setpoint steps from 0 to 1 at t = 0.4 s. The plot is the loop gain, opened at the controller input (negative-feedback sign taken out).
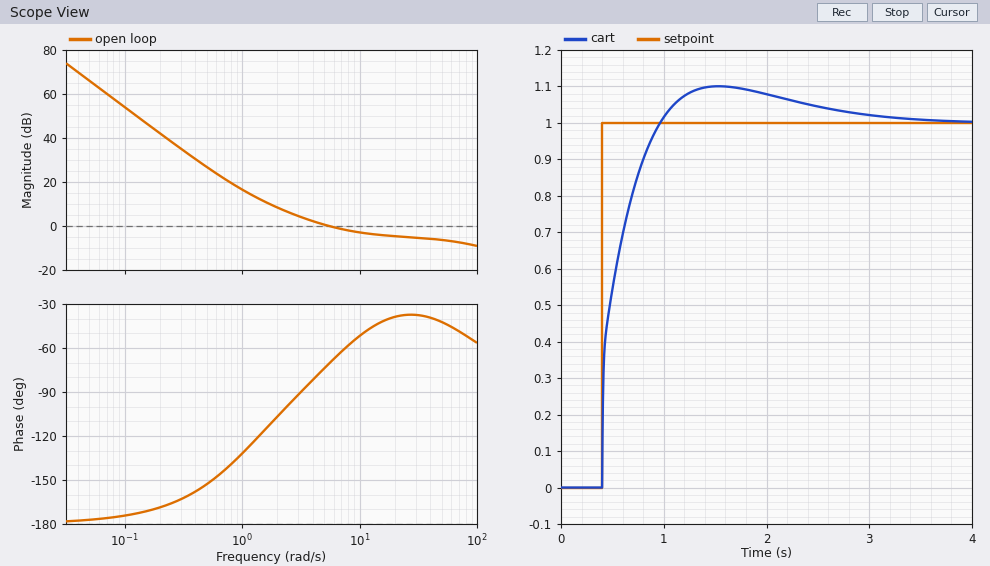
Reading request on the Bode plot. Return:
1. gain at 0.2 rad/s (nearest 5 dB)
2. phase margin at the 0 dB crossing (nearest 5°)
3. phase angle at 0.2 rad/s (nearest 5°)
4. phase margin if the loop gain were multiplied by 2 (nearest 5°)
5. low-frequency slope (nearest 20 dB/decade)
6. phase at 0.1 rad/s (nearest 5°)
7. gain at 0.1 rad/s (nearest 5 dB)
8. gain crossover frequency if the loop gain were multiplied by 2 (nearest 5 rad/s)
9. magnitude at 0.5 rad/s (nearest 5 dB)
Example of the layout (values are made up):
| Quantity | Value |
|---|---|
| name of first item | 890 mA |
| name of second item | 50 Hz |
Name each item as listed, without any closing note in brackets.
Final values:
| Quantity | Value |
|---|---|
| gain at 0.2 rad/s | 40 dB |
| phase margin at the 0 dB crossing | 110° |
| phase angle at 0.2 rad/s | -170° |
| phase margin if the loop gain were multiplied by 2 | 140° |
| low-frequency slope | -40 dB/decade |
| phase at 0.1 rad/s | -175° |
| gain at 0.1 rad/s | 55 dB |
| gain crossover frequency if the loop gain were multiplied by 2 | 45 rad/s |
| magnitude at 0.5 rad/s | 25 dB |
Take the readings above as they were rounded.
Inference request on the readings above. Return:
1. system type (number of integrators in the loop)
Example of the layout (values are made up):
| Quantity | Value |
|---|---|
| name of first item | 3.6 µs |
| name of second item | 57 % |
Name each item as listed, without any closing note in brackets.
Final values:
| Quantity | Value |
|---|---|
| system type | 2 |
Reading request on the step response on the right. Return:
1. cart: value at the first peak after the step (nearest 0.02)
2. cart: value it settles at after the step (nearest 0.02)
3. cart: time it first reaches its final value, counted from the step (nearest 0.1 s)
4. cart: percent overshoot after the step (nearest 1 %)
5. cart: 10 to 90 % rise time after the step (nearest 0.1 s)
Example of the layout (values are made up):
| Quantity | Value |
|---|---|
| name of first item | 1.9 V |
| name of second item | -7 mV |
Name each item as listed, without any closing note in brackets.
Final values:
| Quantity | Value |
|---|---|
| cart: value at the first peak after the step | 1.10 |
| cart: value it settles at after the step | 1.00 |
| cart: time it first reaches its final value, counted from the step | 0.6 s |
| cart: percent overshoot after the step | 10 % |
| cart: 10 to 90 % rise time after the step | 0.4 s |
